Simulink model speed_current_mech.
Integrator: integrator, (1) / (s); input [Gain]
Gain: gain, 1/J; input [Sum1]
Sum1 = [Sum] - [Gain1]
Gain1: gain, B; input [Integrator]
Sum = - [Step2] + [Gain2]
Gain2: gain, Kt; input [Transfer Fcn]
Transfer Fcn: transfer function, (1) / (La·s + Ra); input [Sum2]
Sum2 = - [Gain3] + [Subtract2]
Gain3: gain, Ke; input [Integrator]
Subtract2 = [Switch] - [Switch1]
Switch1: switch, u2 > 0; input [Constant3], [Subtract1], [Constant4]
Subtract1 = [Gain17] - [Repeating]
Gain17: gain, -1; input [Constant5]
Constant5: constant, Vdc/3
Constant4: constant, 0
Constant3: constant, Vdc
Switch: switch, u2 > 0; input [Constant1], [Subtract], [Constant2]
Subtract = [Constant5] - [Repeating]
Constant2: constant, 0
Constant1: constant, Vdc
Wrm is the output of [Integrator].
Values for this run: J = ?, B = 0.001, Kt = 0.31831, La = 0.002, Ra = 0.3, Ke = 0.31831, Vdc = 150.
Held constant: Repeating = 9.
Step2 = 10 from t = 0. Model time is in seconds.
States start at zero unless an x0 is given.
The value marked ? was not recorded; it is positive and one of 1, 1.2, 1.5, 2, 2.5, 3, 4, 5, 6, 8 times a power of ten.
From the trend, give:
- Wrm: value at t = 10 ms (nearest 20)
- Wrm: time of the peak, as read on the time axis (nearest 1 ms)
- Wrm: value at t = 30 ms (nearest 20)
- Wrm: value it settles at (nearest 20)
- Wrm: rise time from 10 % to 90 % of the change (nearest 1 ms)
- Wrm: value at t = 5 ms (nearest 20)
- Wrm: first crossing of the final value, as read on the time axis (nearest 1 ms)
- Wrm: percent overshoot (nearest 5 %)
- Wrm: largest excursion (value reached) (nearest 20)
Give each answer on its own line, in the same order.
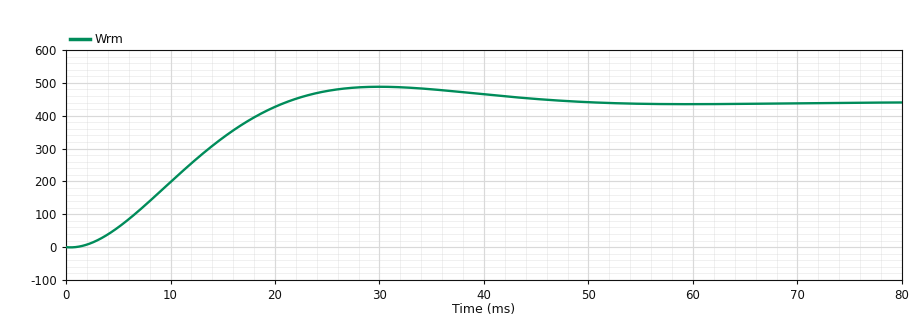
200
30 ms
480
440
14 ms
60
21 ms
10 %
480
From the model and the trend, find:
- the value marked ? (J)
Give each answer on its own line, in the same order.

0.003
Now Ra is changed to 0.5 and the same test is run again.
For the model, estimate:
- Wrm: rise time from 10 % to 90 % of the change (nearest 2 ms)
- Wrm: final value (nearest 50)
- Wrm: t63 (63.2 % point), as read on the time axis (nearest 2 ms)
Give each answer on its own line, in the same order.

24 ms
400
16 ms
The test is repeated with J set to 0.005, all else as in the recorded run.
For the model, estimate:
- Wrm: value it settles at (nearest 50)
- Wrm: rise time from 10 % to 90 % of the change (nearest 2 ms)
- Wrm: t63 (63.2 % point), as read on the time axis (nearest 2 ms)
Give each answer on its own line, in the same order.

450
22 ms
18 ms
